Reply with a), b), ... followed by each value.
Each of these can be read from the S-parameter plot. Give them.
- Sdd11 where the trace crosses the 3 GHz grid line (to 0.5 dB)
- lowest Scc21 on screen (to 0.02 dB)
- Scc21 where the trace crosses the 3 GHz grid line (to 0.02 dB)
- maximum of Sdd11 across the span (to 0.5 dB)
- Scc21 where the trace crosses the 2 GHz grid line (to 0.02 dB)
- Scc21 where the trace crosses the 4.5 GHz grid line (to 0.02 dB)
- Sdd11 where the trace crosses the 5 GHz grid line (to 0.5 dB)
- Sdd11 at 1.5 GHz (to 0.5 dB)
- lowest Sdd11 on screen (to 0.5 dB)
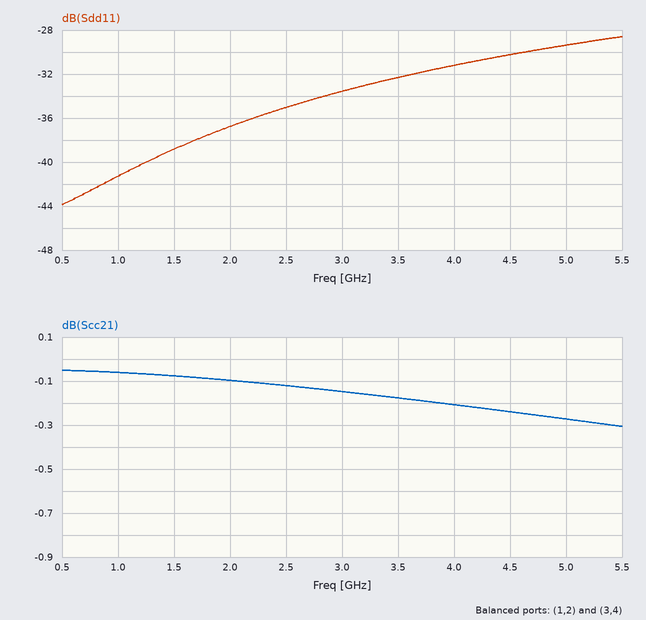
a) -33.5 dB
b) -0.30 dB
c) -0.14 dB
d) -28.5 dB
e) -0.10 dB
f) -0.24 dB
g) -29.5 dB
h) -39.0 dB
i) -44.0 dB
